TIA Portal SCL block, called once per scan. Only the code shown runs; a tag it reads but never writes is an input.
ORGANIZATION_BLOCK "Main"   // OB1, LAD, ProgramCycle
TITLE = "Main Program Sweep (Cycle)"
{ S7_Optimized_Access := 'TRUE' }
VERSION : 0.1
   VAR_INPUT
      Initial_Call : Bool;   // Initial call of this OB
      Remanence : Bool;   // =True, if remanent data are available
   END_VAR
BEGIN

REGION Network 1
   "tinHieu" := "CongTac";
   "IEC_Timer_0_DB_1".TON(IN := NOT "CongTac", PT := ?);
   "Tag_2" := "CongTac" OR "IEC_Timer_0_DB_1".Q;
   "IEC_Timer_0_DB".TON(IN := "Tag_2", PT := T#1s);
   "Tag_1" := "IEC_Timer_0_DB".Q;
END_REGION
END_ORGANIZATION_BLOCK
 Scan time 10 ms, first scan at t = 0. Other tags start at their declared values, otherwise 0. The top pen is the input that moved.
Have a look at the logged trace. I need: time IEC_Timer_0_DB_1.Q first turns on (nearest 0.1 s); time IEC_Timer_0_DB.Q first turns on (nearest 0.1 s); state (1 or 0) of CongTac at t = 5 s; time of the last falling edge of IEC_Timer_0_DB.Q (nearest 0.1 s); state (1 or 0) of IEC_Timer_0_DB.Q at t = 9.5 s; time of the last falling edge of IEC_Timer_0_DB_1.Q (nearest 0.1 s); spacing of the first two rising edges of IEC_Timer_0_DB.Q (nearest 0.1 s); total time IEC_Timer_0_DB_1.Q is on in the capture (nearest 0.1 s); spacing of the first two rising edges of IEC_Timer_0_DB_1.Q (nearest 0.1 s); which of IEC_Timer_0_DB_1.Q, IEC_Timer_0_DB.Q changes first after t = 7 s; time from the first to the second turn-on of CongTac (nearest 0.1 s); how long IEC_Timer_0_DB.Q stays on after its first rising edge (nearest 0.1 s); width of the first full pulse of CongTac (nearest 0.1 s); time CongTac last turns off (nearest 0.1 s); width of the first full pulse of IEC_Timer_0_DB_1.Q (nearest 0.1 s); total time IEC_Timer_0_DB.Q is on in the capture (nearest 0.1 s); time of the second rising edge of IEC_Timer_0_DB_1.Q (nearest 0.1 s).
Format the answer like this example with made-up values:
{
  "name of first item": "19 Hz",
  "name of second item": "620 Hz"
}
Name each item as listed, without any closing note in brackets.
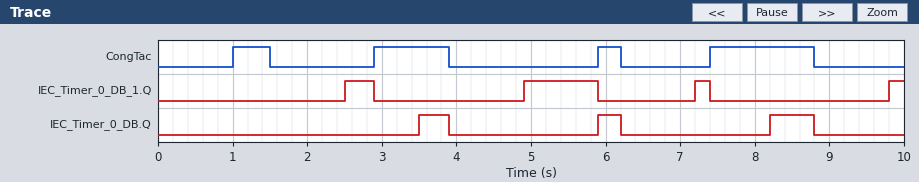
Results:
{
  "time IEC_Timer_0_DB_1.Q first turns on": "2.5 s",
  "time IEC_Timer_0_DB.Q first turns on": "3.5 s",
  "state (1 or 0) of CongTac at t = 5 s": "0",
  "time of the last falling edge of IEC_Timer_0_DB.Q": "8.8 s",
  "state (1 or 0) of IEC_Timer_0_DB.Q at t = 9.5 s": "0",
  "time of the last falling edge of IEC_Timer_0_DB_1.Q": "7.4 s",
  "spacing of the first two rising edges of IEC_Timer_0_DB.Q": "2.4 s",
  "total time IEC_Timer_0_DB_1.Q is on in the capture": "1.8 s",
  "spacing of the first two rising edges of IEC_Timer_0_DB_1.Q": "2.4 s",
  "which of IEC_Timer_0_DB_1.Q, IEC_Timer_0_DB.Q changes first after t = 7 s": "IEC_Timer_0_DB_1.Q",
  "time from the first to the second turn-on of CongTac": "1.9 s",
  "how long IEC_Timer_0_DB.Q stays on after its first rising edge": "0.4 s",
  "width of the first full pulse of CongTac": "0.5 s",
  "time CongTac last turns off": "8.8 s",
  "width of the first full pulse of IEC_Timer_0_DB_1.Q": "0.4 s",
  "total time IEC_Timer_0_DB.Q is on in the capture": "1.3 s",
  "time of the second rising edge of IEC_Timer_0_DB_1.Q": "4.9 s"
}
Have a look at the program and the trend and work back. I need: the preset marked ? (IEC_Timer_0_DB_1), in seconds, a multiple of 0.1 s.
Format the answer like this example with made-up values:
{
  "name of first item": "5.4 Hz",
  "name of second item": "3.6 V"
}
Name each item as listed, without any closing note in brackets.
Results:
{
  "the preset marked ? (IEC_Timer_0_DB_1), in seconds, a multiple of 0.1 s": "1.0 s"
}
